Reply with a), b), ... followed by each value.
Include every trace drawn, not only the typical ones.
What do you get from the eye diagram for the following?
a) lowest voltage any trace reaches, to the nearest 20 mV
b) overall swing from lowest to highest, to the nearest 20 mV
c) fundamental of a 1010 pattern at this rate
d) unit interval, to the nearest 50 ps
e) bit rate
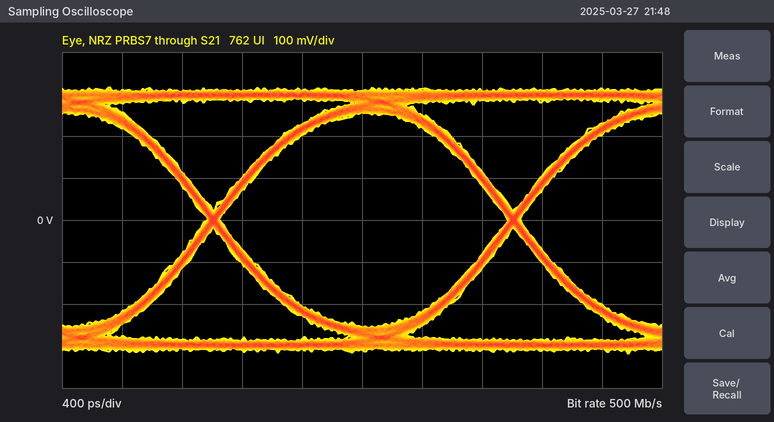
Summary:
a) -320 mV
b) 640 mV
c) 250 MHz
d) 2.00 ns
e) 500 Mb/s
